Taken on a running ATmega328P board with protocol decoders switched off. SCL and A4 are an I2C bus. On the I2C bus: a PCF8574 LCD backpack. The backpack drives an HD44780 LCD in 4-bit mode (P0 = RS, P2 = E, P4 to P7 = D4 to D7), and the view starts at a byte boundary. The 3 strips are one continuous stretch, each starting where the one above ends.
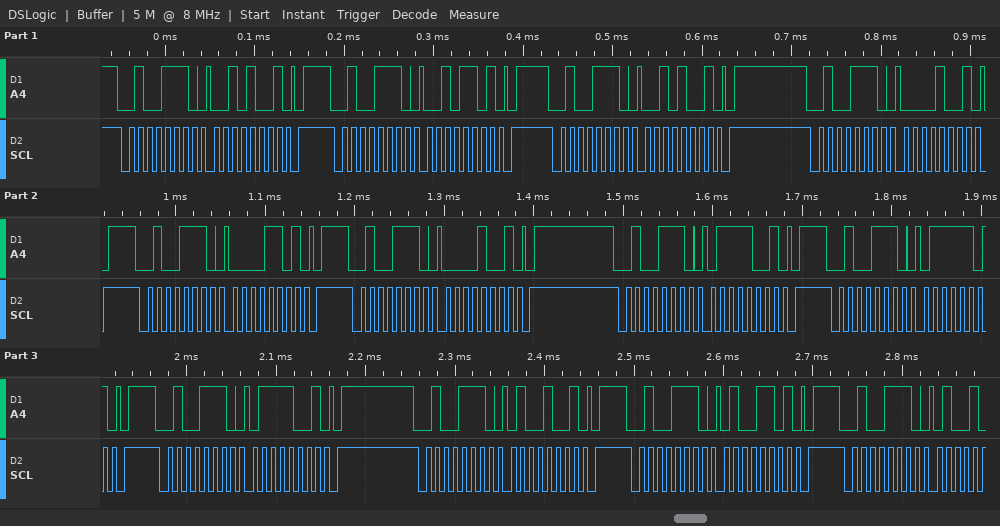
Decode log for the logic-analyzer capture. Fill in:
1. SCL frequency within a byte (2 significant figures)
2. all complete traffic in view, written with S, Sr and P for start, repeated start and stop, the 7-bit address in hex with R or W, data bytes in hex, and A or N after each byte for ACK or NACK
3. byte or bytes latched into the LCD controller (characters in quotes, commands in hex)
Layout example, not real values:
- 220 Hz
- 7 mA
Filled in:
- 100 kHz
- S 27W A 29 A P S 27W A 2D A P S 27W A 29 A P S 27W A 09 A P S 27W A 0D A P S 27W A 09 A P S 27W A 79 A P S 27W A 7D A P S 27W A 79 A P S 27W A 49 A P S 27W A 4D A P S 27W A
- ' '
